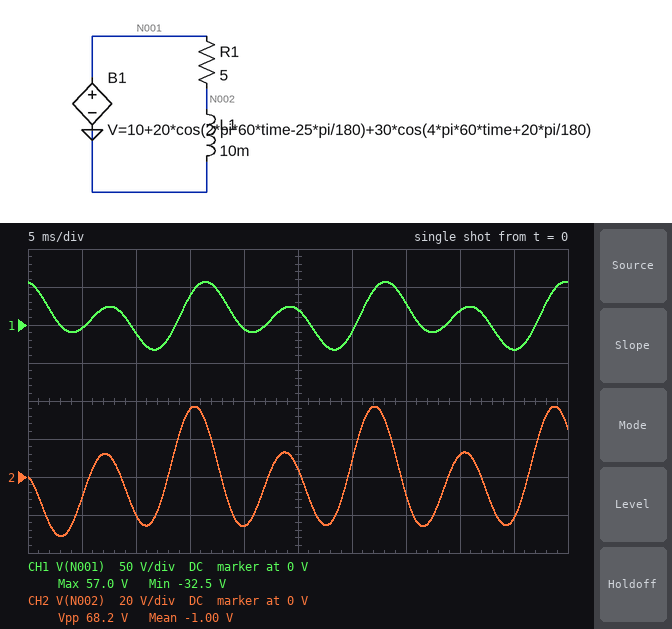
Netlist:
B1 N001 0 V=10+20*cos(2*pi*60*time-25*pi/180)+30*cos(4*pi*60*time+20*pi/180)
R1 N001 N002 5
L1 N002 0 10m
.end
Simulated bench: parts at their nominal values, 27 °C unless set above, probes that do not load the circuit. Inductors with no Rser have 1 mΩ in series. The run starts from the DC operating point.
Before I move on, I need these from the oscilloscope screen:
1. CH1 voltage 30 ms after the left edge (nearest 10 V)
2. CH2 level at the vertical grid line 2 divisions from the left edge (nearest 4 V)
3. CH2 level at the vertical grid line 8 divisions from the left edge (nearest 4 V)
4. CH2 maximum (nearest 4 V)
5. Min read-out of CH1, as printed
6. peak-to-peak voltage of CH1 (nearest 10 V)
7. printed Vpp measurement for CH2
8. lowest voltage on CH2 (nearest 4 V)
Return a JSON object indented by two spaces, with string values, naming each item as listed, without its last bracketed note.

{
  "CH1 voltage 30 ms after the left edge": "-10 V",
  "CH2 level at the vertical grid line 2 divisions from the left edge": "-20 V",
  "CH2 level at the vertical grid line 8 divisions from the left edge": "12 V",
  "CH2 maximum": "36 V",
  "Min read-out of CH1, as printed": "-32.5 V",
  "peak-to-peak voltage of CH1": "90 V",
  "printed Vpp measurement for CH2": "68.2 V",
  "lowest voltage on CH2": "-32 V"
}
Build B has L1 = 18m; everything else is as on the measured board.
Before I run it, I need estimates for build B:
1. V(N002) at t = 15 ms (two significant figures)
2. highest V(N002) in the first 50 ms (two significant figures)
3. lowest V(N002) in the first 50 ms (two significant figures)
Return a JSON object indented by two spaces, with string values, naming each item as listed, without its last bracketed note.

{
  "V(N002) at t = 15 ms": "38 V",
  "highest V(N002) in the first 50 ms": "44 V",
  "lowest V(N002) in the first 50 ms": "-41 V"
}
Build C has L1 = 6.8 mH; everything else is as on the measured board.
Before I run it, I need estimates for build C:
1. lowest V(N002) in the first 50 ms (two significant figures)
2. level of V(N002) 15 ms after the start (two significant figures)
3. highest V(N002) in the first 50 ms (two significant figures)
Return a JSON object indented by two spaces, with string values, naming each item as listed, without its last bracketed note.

{
  "lowest V(N002) in the first 50 ms": "-25 V",
  "level of V(N002) 15 ms after the start": "30 V",
  "highest V(N002) in the first 50 ms": "31 V"
}
